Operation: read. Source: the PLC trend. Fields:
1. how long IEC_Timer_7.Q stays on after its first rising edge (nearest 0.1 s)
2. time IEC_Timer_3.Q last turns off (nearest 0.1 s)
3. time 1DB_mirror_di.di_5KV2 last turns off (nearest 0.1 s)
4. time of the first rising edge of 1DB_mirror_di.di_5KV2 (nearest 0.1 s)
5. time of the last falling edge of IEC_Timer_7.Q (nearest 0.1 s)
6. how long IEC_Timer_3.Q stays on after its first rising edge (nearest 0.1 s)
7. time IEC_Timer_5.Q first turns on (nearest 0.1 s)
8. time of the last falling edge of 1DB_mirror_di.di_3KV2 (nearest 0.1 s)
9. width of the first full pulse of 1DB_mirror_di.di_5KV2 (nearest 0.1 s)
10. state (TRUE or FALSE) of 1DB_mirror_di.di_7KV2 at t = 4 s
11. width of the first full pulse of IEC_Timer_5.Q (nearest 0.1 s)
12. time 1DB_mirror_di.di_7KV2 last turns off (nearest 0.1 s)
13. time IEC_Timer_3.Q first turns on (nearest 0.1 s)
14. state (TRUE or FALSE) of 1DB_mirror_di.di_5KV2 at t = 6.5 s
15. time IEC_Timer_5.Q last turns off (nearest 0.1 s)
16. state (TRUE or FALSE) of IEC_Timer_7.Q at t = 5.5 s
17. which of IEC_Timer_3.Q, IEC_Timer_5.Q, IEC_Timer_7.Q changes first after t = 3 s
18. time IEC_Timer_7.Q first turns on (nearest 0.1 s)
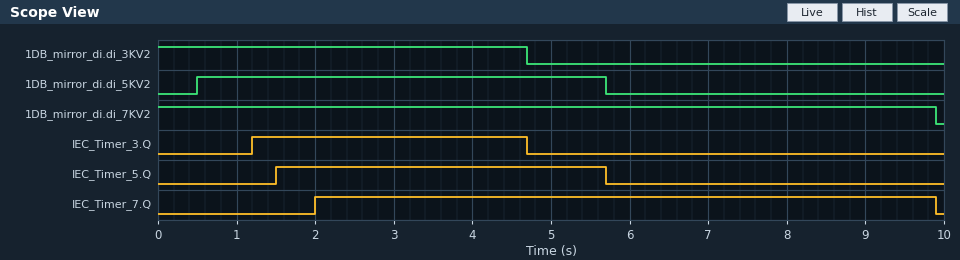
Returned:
7.9 s
4.7 s
5.7 s
0.5 s
9.9 s
3.5 s
1.5 s
4.7 s
5.2 s
TRUE
4.2 s
9.9 s
1.2 s
FALSE
5.7 s
TRUE
IEC_Timer_3.Q
2.0 s
